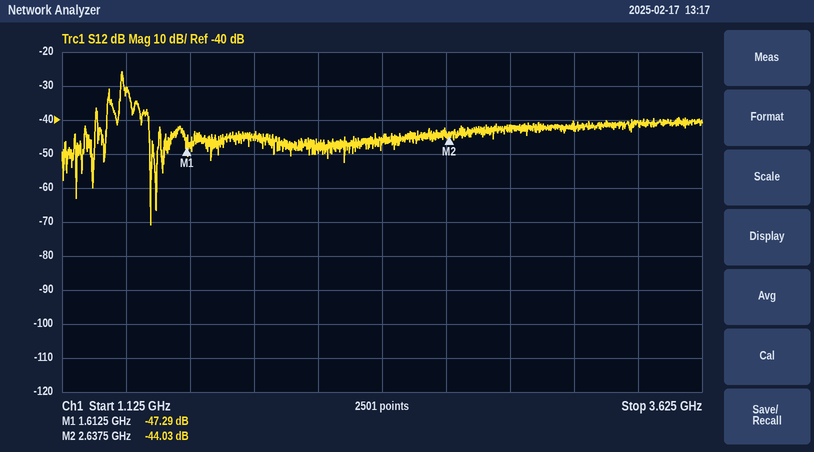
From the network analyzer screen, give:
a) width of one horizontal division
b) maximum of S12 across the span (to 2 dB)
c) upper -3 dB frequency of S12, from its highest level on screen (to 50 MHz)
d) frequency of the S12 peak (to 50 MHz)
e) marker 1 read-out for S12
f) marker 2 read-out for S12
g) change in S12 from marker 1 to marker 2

250 MHz
-26 dB
1.35 GHz
1.35 GHz
-47.29 dB
-44.03 dB
3.26 dB
